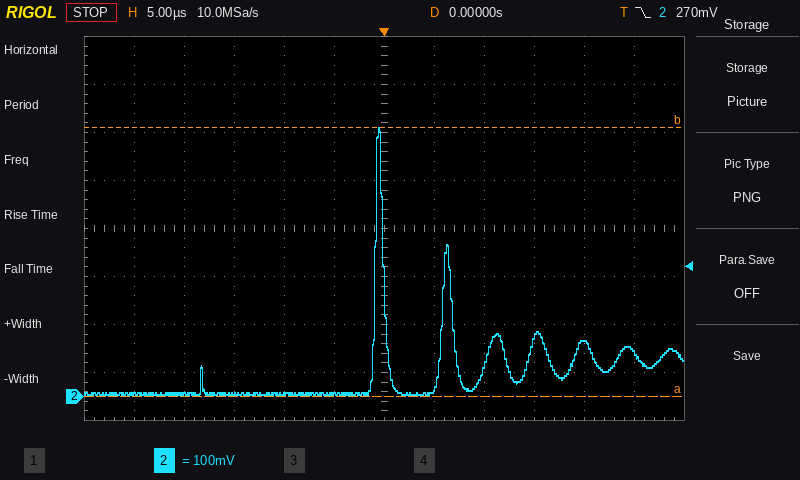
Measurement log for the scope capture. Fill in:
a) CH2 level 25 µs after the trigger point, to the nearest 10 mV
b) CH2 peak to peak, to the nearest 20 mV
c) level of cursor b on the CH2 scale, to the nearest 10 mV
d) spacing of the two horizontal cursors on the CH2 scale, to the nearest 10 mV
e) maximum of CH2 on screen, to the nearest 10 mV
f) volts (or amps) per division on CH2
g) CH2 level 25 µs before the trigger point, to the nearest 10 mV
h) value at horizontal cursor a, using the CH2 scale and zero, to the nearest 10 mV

90 mV
560 mV
560 mV
560 mV
560 mV
100 mV
10 mV
0 mV
